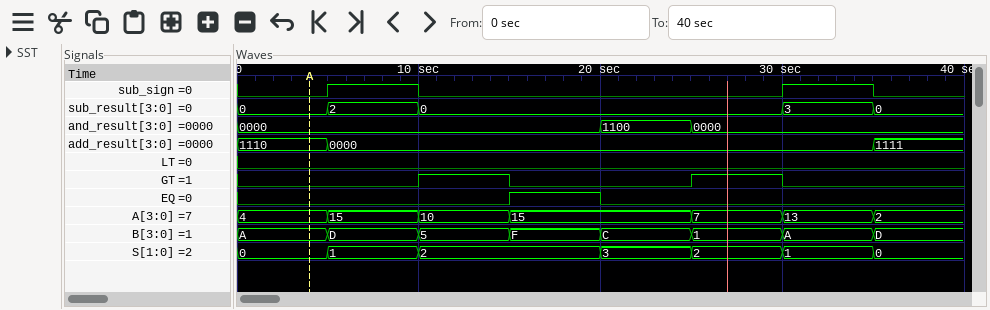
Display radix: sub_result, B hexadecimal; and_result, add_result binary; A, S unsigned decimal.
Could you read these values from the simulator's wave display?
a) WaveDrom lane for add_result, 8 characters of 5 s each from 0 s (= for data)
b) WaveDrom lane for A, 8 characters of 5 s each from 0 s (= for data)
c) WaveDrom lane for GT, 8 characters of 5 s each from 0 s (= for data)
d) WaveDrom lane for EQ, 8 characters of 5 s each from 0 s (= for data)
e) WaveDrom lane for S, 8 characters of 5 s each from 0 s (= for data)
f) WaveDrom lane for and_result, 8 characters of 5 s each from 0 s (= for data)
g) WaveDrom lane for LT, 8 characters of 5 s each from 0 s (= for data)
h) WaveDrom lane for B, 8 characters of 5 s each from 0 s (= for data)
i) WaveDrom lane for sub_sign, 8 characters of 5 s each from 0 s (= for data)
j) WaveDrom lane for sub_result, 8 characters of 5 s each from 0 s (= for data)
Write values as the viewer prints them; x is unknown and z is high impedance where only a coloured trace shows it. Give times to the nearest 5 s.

{name: 'add_result', wave: '==.....=', data: '1110 0000 1111'}
{name: 'A', wave: '====.===', data: '4 15 10 15 7 13 2'}
{name: 'GT', wave: '0.10.10.'}
{name: 'EQ', wave: '0..10...'}
{name: 'S', wave: '===.====', data: '0 1 2 3 2 1 0'}
{name: 'and_result', wave: '=...==..', data: '0000 1100 0000'}
{name: 'LT', wave: '0.......'}
{name: 'B', wave: '========', data: 'A D 5 F C 1 A D'}
{name: 'sub_sign', wave: '010...10'}
{name: 'sub_result', wave: '===...==', data: '0 2 0 3 0'}
